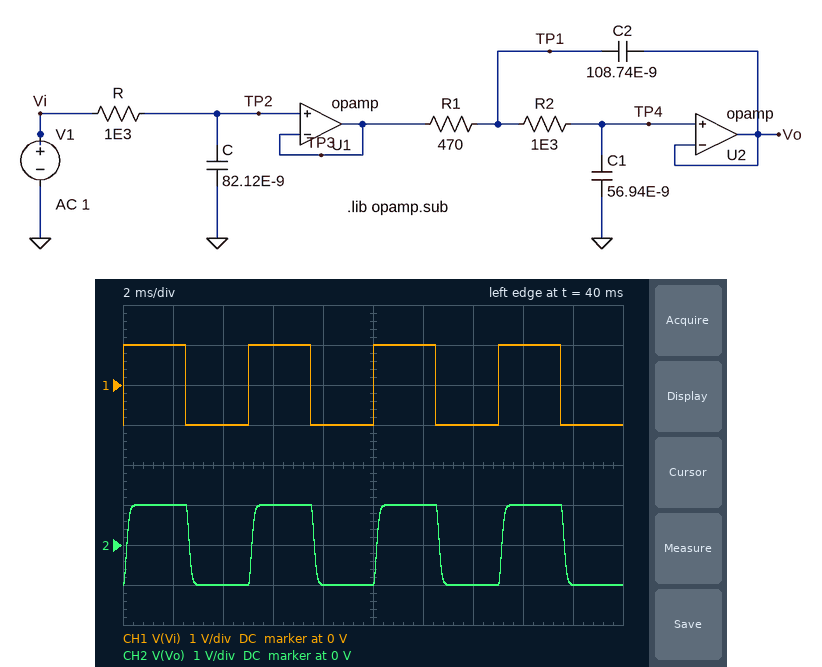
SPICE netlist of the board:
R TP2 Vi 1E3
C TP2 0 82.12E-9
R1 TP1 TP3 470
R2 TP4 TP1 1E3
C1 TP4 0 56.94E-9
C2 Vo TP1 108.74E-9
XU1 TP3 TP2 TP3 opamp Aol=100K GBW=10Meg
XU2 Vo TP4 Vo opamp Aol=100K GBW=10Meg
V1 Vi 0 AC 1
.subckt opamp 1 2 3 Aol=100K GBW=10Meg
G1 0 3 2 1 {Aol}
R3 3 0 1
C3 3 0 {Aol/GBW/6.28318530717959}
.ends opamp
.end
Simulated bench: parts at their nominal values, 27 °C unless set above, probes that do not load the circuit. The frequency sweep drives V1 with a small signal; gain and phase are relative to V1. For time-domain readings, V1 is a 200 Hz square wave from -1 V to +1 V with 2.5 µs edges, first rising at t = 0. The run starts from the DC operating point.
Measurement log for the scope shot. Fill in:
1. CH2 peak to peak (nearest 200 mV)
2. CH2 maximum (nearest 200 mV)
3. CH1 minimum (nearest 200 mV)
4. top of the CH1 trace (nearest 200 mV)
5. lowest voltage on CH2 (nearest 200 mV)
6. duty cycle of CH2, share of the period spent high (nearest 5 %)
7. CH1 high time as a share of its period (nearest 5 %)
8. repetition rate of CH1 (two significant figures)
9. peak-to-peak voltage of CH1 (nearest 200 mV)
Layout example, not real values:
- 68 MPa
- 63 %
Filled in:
- 2.0 V
- 1.0 V
- -1.0 V
- 1.0 V
- -1.0 V
- 50 %
- 50 %
- 200 Hz
- 2.0 V
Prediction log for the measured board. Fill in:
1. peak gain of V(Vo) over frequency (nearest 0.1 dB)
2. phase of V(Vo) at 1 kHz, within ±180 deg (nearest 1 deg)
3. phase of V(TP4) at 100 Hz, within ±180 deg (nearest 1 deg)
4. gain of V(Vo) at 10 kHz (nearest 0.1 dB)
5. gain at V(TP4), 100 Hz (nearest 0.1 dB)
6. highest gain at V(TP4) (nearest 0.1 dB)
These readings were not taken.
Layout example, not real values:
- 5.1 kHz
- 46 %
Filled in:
- 0 dB
- -58 deg
- -6 deg
- -35.8 dB
- 0 dB
- 0 dB
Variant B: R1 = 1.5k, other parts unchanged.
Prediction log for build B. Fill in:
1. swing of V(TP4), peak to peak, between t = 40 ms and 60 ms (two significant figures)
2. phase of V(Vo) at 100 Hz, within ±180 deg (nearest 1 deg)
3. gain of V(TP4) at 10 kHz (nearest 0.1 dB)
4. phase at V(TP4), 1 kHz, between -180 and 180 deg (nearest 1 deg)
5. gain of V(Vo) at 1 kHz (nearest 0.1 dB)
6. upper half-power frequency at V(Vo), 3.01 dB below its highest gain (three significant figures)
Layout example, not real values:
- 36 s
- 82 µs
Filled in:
- 2.1 V
- -8 deg
- -45.7 dB
- -82 deg
- -1.8 dB
- 1.24 kHz
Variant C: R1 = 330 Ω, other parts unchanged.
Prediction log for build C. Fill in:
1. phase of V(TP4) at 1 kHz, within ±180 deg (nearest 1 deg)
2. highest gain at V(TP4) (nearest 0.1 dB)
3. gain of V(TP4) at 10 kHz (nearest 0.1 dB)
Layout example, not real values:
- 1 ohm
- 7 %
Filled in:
- -55 deg
- 0 dB
- -33.0 dB
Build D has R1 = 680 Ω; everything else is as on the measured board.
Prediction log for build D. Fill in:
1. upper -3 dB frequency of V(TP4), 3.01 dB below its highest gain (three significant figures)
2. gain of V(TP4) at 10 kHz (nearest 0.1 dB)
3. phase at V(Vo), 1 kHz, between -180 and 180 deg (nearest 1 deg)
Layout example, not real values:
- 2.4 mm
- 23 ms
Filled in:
- 1.54 kHz
- -38.9 dB
- -63 deg
